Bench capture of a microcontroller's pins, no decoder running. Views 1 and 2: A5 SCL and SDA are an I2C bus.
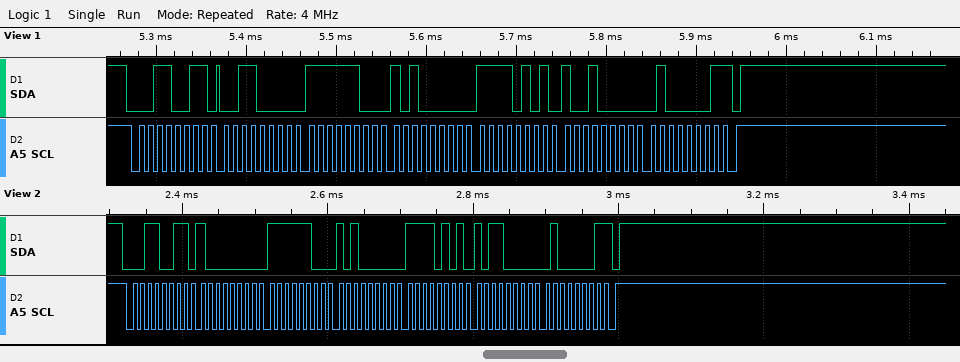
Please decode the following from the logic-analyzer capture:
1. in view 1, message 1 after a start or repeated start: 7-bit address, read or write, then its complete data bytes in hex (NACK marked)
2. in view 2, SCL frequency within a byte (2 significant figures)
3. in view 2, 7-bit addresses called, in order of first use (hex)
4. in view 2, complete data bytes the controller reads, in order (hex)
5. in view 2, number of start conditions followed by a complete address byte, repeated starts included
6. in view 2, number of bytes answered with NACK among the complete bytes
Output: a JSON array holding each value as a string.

["0x19 read: 30 FC A0 F5 90 41 NACK", "100 kHz", "0x19", "80 FC A0 F5 B0 41", "1", "1"]
